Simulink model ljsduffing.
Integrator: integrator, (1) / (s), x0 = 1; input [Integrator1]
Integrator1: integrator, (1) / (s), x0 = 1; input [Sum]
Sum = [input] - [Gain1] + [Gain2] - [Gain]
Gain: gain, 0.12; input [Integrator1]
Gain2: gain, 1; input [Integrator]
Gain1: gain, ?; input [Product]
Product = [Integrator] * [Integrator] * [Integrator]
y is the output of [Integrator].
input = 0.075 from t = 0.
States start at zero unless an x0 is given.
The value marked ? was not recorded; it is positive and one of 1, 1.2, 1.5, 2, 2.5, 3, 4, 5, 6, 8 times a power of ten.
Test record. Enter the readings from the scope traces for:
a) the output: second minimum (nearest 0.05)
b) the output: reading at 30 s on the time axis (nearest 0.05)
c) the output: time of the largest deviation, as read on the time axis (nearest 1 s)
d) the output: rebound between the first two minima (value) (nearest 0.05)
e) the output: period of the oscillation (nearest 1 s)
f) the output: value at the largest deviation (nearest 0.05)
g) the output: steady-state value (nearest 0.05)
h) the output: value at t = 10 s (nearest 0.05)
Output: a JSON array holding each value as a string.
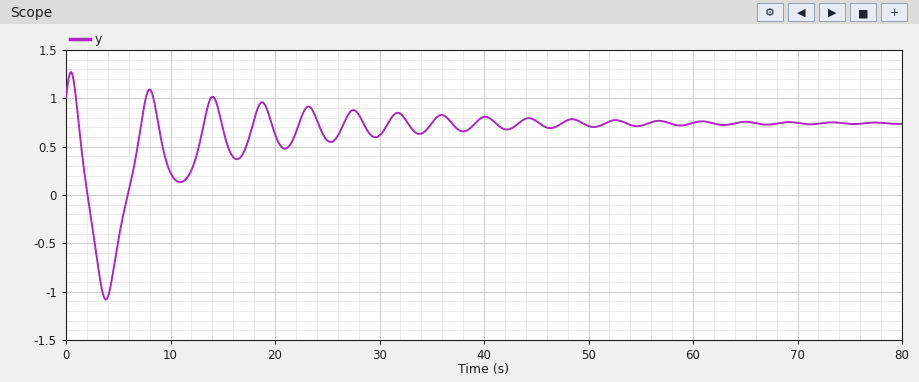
["0.15", "0.60", "4 s", "1.10", "7 s", "-1.10", "0.75", "0.25"]
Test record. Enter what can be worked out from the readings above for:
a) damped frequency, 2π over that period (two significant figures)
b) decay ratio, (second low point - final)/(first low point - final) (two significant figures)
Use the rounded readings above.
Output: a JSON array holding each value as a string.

["0.90 rad/s", "0.32"]
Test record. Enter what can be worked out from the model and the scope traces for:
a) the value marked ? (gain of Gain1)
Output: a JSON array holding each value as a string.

["2"]
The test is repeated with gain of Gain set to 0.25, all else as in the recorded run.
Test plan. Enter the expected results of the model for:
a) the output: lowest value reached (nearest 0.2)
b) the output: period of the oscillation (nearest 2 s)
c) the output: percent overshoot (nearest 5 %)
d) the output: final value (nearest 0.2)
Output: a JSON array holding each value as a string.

["-1.0", "6 s", "15 %", "-0.6"]
